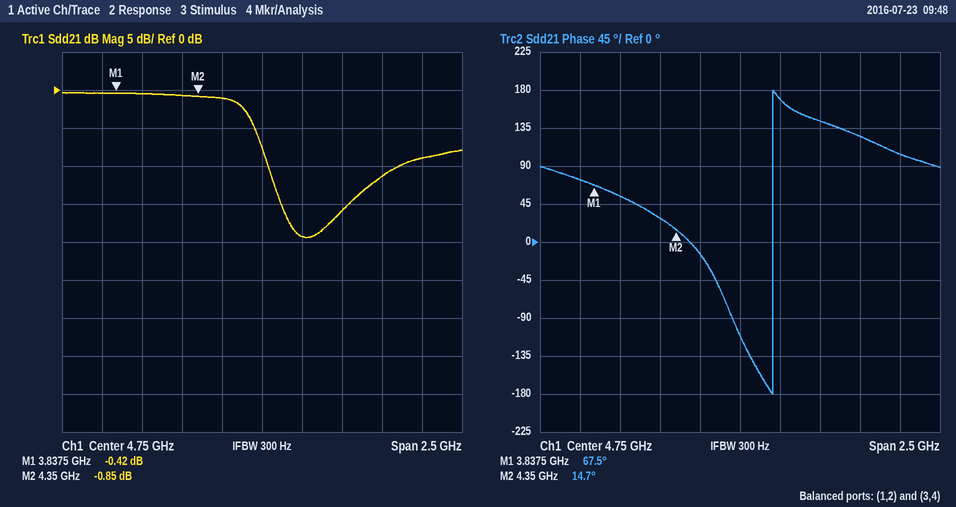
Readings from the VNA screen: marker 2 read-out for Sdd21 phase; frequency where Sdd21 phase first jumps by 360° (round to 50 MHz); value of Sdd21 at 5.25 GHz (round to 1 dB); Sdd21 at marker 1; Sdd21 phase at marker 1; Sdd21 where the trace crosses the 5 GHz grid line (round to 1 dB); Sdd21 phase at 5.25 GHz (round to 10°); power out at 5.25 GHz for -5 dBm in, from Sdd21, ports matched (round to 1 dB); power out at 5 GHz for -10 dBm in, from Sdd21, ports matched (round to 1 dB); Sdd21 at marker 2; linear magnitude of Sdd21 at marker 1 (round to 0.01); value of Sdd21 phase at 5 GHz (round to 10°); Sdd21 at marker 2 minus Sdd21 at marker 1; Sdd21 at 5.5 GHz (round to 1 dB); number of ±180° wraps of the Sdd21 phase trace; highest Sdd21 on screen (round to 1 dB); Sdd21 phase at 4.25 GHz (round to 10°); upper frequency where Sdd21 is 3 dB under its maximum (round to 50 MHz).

14.7°
4.95 GHz
-16 dB
-0.42 dB
67.5°
-19 dB
140°
-21 dBm
-29 dBm
-0.85 dB
0.95
170°
-0.43 dB
-11 dB
1
0 dB
30°
4.65 GHz
